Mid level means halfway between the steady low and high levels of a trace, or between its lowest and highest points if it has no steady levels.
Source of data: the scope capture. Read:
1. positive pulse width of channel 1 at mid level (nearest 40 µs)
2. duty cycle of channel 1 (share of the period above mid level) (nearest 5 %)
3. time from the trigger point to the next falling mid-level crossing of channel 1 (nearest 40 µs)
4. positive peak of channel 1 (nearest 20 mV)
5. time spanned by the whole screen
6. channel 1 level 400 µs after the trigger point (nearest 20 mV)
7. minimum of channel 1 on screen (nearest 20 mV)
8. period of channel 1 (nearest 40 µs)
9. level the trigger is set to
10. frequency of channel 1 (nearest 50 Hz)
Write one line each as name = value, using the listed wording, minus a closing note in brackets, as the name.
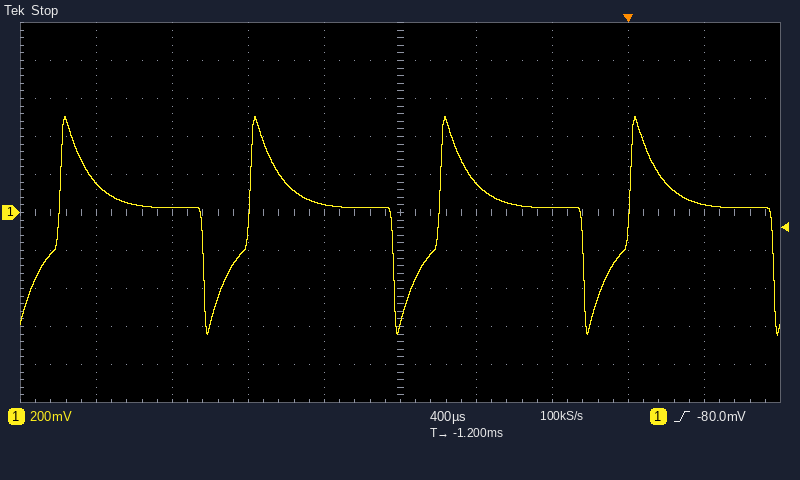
positive pulse width of channel 1 at mid level = 760 µs
duty cycle of channel 1 (share of the period above mid level) = 75 %
time from the trigger point to the next falling mid-level crossing of channel 1 = 760 µs
positive peak of channel 1 = 500 mV
time spanned by the whole screen = 4 ms
channel 1 level 400 µs after the trigger point = 40 mV
minimum of channel 1 on screen = -640 mV
period of channel 1 = 1.00 ms
level the trigger is set to = -80.0 mV
frequency of channel 1 = 1.00 kHz
